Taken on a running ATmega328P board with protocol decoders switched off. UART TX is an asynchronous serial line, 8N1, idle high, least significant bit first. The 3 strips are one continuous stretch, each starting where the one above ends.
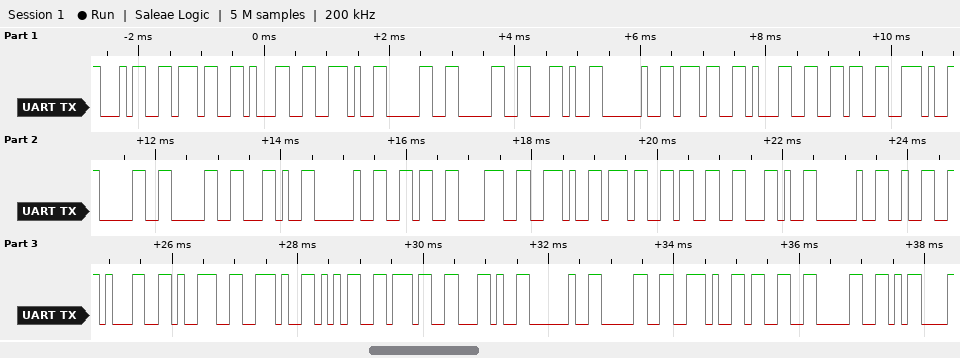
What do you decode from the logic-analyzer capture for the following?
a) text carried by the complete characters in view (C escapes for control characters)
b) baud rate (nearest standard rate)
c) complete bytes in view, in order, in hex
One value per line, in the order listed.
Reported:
"471.00, 716.00, 68.73, 219.57, 0.30\r"
9600 baud
34 37 31 2E 30 30 2C 20 37 31 36 2E 30 30 2C 20 36 38 2E 37 33 2C 20 32 31 39 2E 35 37 2C 20 30 2E 33 30 0D
